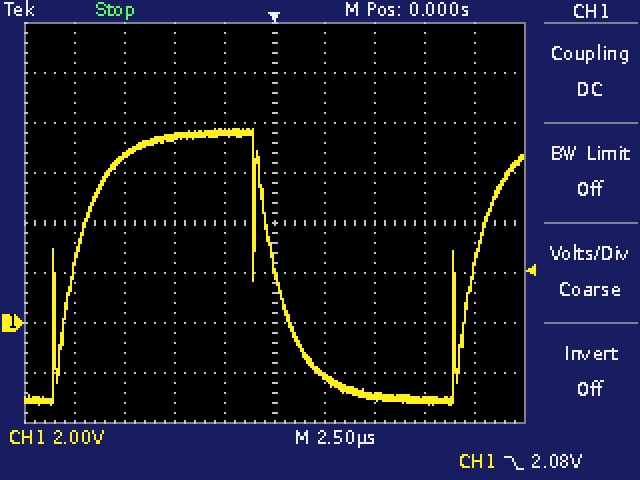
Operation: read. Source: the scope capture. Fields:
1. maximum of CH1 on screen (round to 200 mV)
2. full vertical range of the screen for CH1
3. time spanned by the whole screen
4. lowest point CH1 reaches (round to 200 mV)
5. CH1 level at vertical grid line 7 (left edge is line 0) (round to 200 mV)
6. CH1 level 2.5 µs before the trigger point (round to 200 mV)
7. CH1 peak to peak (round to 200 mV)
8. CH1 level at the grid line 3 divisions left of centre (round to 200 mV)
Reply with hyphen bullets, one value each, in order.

- 7.8 V
- 16 V
- 25 µs
- -3.2 V
- -3.0 V
- 7.6 V
- 11.0 V
- 6.6 V
